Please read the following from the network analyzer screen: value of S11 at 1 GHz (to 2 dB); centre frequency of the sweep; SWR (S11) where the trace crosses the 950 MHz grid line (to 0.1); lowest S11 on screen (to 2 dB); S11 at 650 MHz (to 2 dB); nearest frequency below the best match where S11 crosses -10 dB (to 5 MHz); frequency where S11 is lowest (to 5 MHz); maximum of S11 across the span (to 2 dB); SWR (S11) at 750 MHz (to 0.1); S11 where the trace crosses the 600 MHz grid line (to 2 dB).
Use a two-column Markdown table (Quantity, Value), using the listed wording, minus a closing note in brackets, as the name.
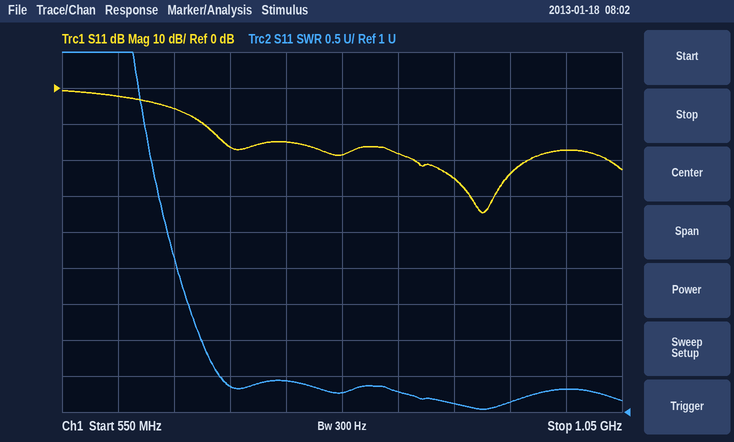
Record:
| Quantity | Value |
|---|---|
| value of S11 at 1 GHz | -18 dB |
| centre frequency of the sweep | 800 MHz |
| SWR (S11) where the trace crosses the 950 MHz grid line | 1.1 |
| lowest S11 on screen | -34 dB |
| S11 at 650 MHz | -6 dB |
| nearest frequency below the best match where S11 crosses -10 dB | 675 MHz |
| frequency where S11 is lowest | 925 MHz |
| maximum of S11 across the span | 0 dB |
| SWR (S11) at 750 MHz | 1.4 |
| S11 where the trace crosses the 600 MHz grid line | -2 dB |
